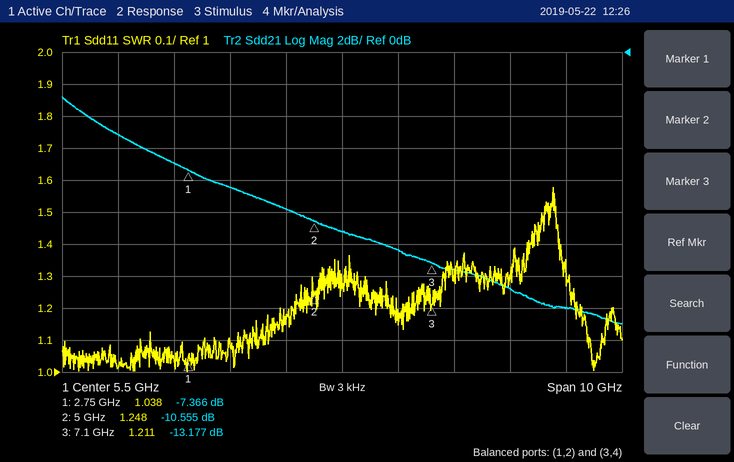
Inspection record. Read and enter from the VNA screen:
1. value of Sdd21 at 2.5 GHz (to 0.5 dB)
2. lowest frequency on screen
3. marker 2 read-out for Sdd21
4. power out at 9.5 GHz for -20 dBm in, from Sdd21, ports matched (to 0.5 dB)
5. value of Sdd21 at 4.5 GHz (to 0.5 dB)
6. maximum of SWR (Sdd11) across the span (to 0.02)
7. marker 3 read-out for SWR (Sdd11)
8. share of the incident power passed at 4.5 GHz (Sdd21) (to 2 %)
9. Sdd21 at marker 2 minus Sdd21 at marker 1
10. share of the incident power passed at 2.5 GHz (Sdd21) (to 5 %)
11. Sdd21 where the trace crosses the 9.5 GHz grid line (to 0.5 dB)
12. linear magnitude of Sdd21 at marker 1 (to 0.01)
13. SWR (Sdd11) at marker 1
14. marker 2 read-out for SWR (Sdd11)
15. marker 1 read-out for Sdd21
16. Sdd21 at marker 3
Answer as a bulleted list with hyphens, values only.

- -7.0 dB
- 500 MHz
- -10.555 dB
- -36.0 dBm
- -10.0 dB
- 1.58
- 1.211
- 10 %
- -3.189 dB
- 20 %
- -16.0 dB
- 0.43
- 1.038
- 1.248
- -7.366 dB
- -13.177 dB
